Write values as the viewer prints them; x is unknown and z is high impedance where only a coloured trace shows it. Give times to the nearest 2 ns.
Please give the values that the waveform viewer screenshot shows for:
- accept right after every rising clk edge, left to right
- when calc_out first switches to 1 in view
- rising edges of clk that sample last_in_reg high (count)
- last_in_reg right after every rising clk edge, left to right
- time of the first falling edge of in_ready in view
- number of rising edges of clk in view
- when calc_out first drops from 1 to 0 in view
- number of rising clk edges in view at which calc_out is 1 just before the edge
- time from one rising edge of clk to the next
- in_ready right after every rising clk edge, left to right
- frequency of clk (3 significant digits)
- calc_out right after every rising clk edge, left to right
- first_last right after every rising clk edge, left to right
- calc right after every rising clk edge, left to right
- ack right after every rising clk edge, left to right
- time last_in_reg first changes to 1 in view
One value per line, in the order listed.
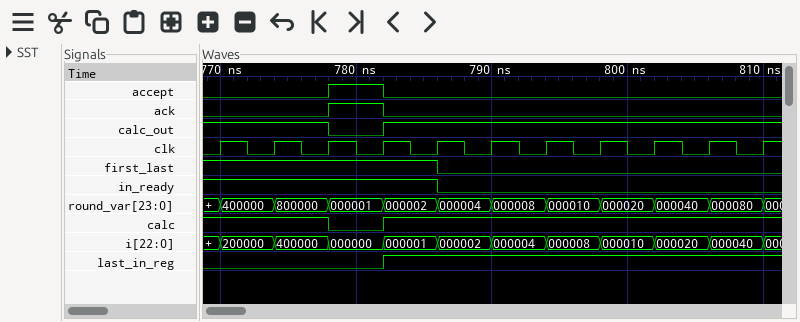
0 0 1 0 0 0 0 0 0 0 0
782 ns
7
0 0 0 1 1 1 1 1 1 1 1
786 ns
11
778 ns
10
4 ns
1 1 1 1 0 0 0 0 0 0 0
250 MHz
1 1 0 1 1 1 1 1 1 1 1
1 1 1 1 0 0 0 0 0 0 0
1 1 0 1 1 1 1 1 1 1 1
0 0 1 0 0 0 0 0 0 0 0
782 ns
